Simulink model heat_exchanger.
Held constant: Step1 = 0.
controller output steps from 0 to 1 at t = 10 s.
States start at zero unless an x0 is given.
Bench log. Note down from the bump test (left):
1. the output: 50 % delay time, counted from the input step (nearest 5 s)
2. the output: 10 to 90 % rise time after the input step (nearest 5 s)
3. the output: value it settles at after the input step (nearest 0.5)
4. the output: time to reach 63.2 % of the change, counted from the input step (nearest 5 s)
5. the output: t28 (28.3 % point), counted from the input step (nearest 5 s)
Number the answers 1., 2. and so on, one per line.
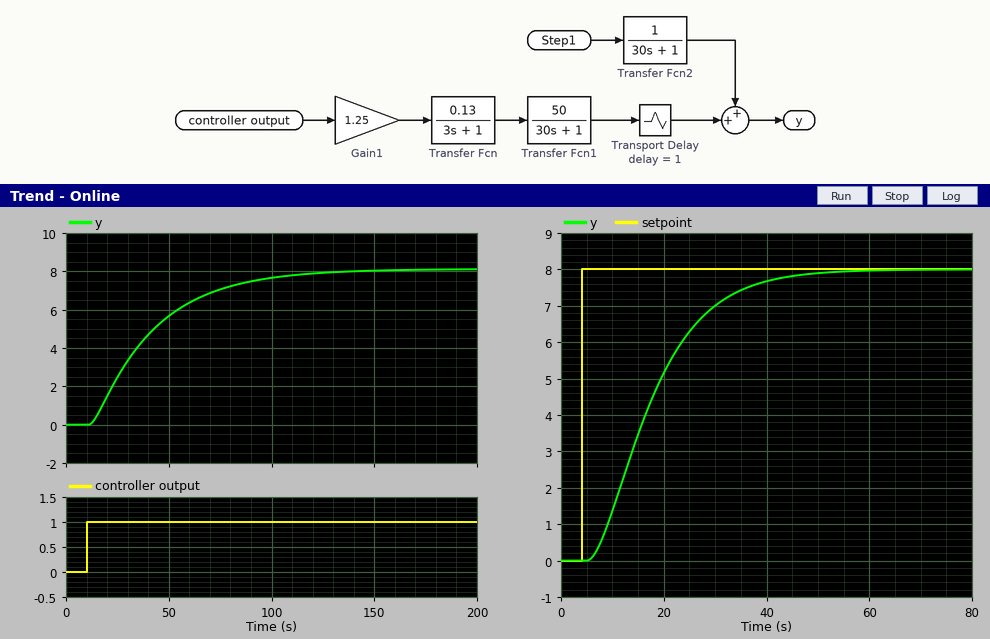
1. 25 s
2. 65 s
3. 8.0
4. 35 s
5. 15 s
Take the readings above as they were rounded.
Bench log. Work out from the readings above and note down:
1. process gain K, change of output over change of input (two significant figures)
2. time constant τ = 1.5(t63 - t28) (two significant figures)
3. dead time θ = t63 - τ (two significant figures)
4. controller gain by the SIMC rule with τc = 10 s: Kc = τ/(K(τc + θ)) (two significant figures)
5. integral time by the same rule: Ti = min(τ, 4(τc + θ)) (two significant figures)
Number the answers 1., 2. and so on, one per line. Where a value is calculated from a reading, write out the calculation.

1. (8 - 0) / 1 = 8.0
2. 1.5 × (35 - 15) = 30 s
3. 35 - 30 = 5.0 s
4. 30 / (8 × (10 + 5)) = 0.25
5. min(30, 4 × (10 + 5)) = 30 s
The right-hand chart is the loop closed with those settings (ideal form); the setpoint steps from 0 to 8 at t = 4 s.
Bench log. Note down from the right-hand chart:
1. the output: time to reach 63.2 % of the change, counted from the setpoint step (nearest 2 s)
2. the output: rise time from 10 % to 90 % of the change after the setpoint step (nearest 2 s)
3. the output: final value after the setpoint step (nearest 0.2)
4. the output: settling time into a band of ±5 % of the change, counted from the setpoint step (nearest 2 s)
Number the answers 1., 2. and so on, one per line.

1. 16 s
2. 24 s
3. 8.0
4. 34 s
